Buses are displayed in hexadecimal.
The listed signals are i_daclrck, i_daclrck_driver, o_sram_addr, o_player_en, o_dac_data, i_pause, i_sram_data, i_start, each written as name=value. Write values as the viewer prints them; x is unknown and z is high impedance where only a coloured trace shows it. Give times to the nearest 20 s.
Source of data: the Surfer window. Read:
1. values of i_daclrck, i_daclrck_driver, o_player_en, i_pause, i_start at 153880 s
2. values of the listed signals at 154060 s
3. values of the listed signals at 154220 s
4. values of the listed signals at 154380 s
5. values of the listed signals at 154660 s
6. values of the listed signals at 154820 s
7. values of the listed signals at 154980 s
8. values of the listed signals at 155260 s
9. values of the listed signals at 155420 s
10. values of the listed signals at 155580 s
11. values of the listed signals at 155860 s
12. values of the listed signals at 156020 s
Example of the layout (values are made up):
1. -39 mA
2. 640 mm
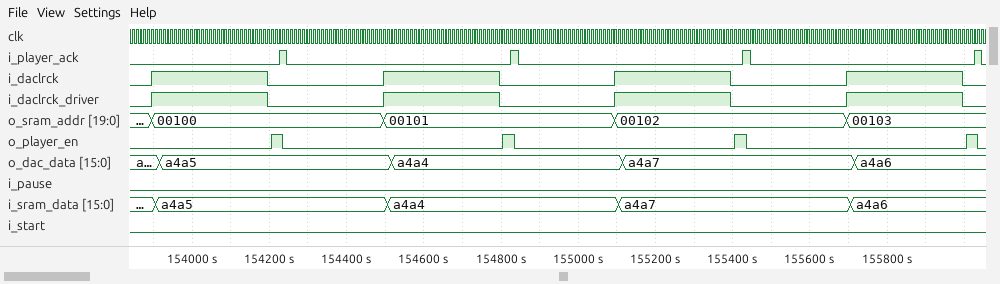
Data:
1. i_daclrck=0, i_daclrck_driver=0, o_player_en=0, i_pause=0, i_start=0
2. i_daclrck=1, i_daclrck_driver=1, o_sram_addr=00100, o_player_en=0, o_dac_data=a4a5, i_pause=0, i_sram_data=a4a5, i_start=0
3. i_daclrck=0, i_daclrck_driver=0, o_sram_addr=00100, o_player_en=1, o_dac_data=a4a5, i_pause=0, i_sram_data=a4a5, i_start=0
4. i_daclrck=0, i_daclrck_driver=0, o_sram_addr=00100, o_player_en=0, o_dac_data=a4a5, i_pause=0, i_sram_data=a4a5, i_start=0
5. i_daclrck=1, i_daclrck_driver=1, o_sram_addr=00101, o_player_en=0, o_dac_data=a4a4, i_pause=0, i_sram_data=a4a4, i_start=0
6. i_daclrck=0, i_daclrck_driver=0, o_sram_addr=00101, o_player_en=1, o_dac_data=a4a4, i_pause=0, i_sram_data=a4a4, i_start=0
7. i_daclrck=0, i_daclrck_driver=0, o_sram_addr=00101, o_player_en=0, o_dac_data=a4a4, i_pause=0, i_sram_data=a4a4, i_start=0
8. i_daclrck=1, i_daclrck_driver=1, o_sram_addr=00102, o_player_en=0, o_dac_data=a4a7, i_pause=0, i_sram_data=a4a7, i_start=0
9. i_daclrck=0, i_daclrck_driver=0, o_sram_addr=00102, o_player_en=1, o_dac_data=a4a7, i_pause=0, i_sram_data=a4a7, i_start=0
10. i_daclrck=0, i_daclrck_driver=0, o_sram_addr=00102, o_player_en=0, o_dac_data=a4a7, i_pause=0, i_sram_data=a4a7, i_start=0
11. i_daclrck=1, i_daclrck_driver=1, o_sram_addr=00103, o_player_en=0, o_dac_data=a4a6, i_pause=0, i_sram_data=a4a6, i_start=0
12. i_daclrck=0, i_daclrck_driver=0, o_sram_addr=00103, o_player_en=1, o_dac_data=a4a6, i_pause=0, i_sram_data=a4a6, i_start=0
